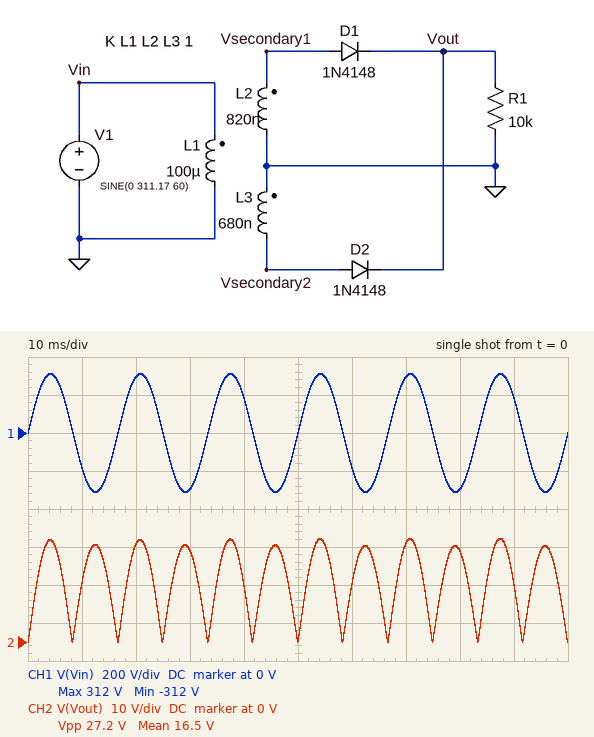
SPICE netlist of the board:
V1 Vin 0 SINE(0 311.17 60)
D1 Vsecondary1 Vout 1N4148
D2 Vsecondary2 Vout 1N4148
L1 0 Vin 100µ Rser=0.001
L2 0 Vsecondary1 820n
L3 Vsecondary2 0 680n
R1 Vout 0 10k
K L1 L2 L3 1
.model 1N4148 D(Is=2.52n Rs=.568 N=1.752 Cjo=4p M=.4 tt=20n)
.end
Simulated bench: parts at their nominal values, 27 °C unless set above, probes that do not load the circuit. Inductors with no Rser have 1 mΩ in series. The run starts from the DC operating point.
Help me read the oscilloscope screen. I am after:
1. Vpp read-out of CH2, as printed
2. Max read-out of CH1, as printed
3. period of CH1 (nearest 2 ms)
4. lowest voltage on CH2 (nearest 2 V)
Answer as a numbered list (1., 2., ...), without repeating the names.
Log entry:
1. 27.2 V
2. 312 V
3. 16 ms
4. 0 V
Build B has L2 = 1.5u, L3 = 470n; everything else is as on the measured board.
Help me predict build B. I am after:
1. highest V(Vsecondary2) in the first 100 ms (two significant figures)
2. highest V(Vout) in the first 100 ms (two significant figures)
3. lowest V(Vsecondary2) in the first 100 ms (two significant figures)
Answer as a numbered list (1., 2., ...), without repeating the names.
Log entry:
1. 22 V
2. 37 V
3. -21 V
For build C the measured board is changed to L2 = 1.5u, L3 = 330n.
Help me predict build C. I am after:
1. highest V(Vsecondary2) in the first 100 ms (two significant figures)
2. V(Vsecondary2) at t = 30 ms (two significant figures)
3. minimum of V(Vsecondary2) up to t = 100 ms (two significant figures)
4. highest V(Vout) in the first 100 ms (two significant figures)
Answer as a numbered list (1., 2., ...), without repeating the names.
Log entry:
1. 18 V
2. 17 V
3. -18 V
4. 37 V
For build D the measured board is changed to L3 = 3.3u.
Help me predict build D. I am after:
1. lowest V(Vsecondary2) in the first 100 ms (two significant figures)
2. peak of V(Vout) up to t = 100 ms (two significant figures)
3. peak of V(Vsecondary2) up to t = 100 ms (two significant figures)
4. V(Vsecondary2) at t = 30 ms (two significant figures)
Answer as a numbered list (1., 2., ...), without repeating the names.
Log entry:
1. -56 V
2. 57 V
3. 58 V
4. 54 V
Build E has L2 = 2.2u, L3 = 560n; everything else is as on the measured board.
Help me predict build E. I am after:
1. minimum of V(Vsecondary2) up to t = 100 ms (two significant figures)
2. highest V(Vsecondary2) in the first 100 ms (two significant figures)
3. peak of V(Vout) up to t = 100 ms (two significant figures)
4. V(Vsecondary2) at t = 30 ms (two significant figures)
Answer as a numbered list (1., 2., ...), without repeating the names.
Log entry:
1. -23 V
2. 24 V
3. 45 V
4. 22 V
